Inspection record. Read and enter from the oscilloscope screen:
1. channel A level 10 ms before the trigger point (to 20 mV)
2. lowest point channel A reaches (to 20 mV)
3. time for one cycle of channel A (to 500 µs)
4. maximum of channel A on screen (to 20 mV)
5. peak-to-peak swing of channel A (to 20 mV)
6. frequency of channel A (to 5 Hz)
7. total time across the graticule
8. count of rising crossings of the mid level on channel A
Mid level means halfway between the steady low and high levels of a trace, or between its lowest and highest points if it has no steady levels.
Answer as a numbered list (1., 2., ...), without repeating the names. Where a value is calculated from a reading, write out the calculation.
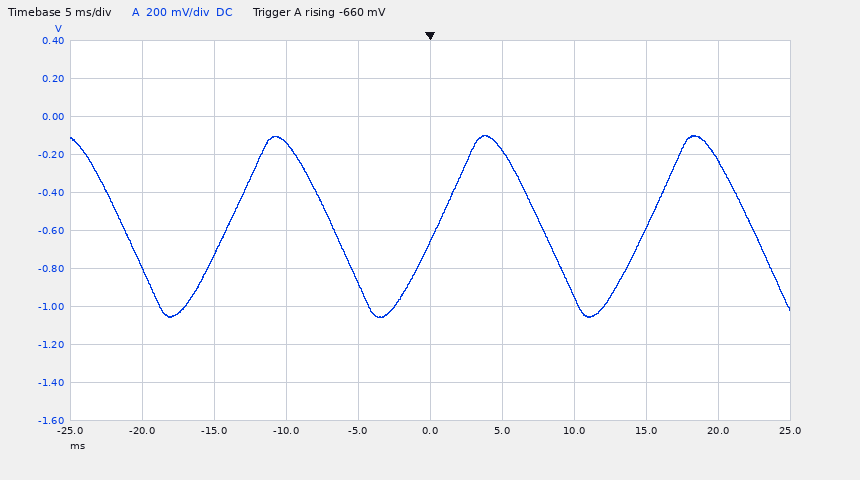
1. -140 mV
2. -1.06 V
3. 14.5 ms
4. -100 mV
5. -100 mV − (-1.06 V) = 960 mV
6. 1 / 14.5 ms ≈ 69.0 Hz, so 70 Hz to the nearest 5 Hz
7. 50 ms
8. 3
